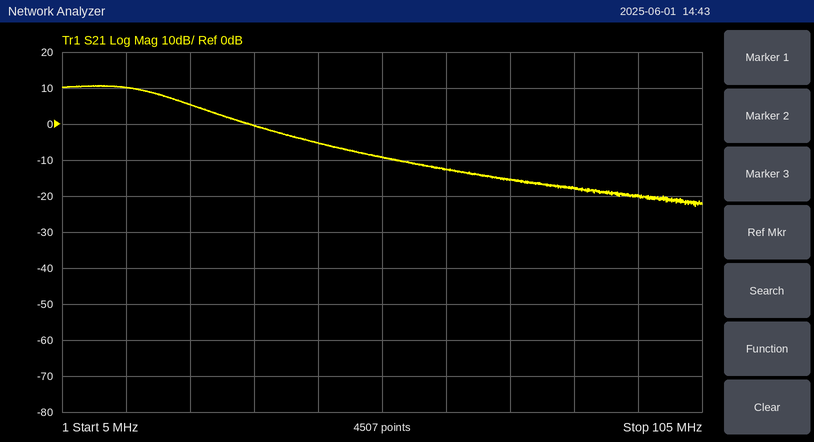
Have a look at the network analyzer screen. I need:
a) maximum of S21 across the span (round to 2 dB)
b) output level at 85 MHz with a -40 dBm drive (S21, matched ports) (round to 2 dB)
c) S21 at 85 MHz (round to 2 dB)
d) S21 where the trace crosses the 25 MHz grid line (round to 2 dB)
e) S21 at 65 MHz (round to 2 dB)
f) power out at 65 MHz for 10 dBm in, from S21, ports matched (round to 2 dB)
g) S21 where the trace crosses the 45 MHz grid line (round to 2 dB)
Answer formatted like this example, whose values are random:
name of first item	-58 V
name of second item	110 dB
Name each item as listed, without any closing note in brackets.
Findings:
maximum of S21 across the span	10 dB
output level at 85 MHz with a -40 dBm drive (S21, matched ports)	-58 dBm
S21 at 85 MHz	-18 dB
S21 where the trace crosses the 25 MHz grid line	6 dB
S21 at 65 MHz	-12 dB
power out at 65 MHz for 10 dBm in, from S21, ports matched	-2 dBm
S21 where the trace crosses the 45 MHz grid line	-6 dB
